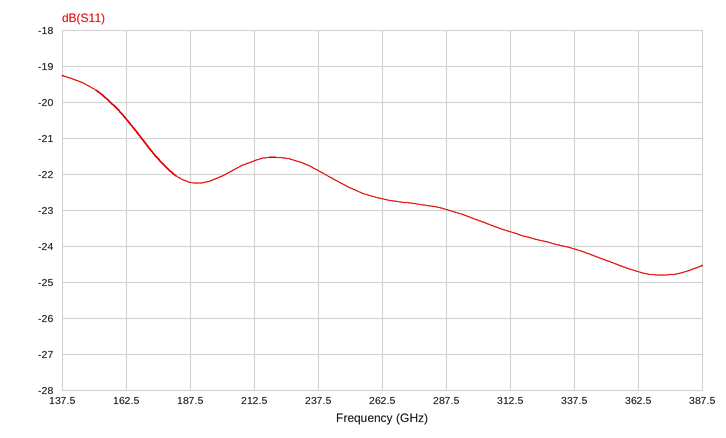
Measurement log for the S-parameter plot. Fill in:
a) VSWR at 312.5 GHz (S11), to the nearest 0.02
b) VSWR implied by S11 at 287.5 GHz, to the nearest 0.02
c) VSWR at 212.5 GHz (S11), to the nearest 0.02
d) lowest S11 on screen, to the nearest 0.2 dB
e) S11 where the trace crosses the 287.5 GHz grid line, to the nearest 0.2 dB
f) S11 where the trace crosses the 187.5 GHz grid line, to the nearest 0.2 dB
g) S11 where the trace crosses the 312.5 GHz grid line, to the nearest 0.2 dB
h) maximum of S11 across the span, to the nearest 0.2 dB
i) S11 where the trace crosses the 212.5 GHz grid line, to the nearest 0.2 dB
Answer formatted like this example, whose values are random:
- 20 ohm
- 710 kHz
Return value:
- 1.14
- 1.16
- 1.18
- -24.8 dB
- -23.0 dB
- -22.2 dB
- -23.6 dB
- -19.2 dB
- -21.6 dB
